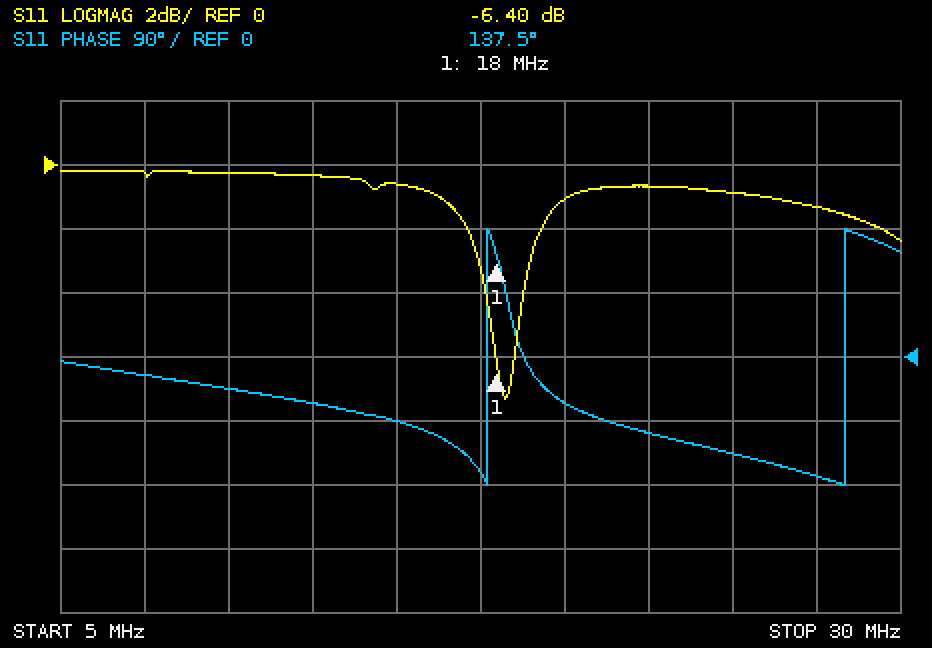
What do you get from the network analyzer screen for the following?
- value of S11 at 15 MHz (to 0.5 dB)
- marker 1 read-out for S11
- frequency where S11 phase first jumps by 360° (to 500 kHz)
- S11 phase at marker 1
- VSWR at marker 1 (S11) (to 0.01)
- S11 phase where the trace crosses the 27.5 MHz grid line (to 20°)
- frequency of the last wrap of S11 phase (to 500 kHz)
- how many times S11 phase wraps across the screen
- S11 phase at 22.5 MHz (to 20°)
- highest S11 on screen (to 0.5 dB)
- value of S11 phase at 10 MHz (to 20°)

-0.5 dB
-6.40 dB
17.5 MHz
137.5°
2.84
-160°
28.5 MHz
2
-100°
0.0 dB
-40°
